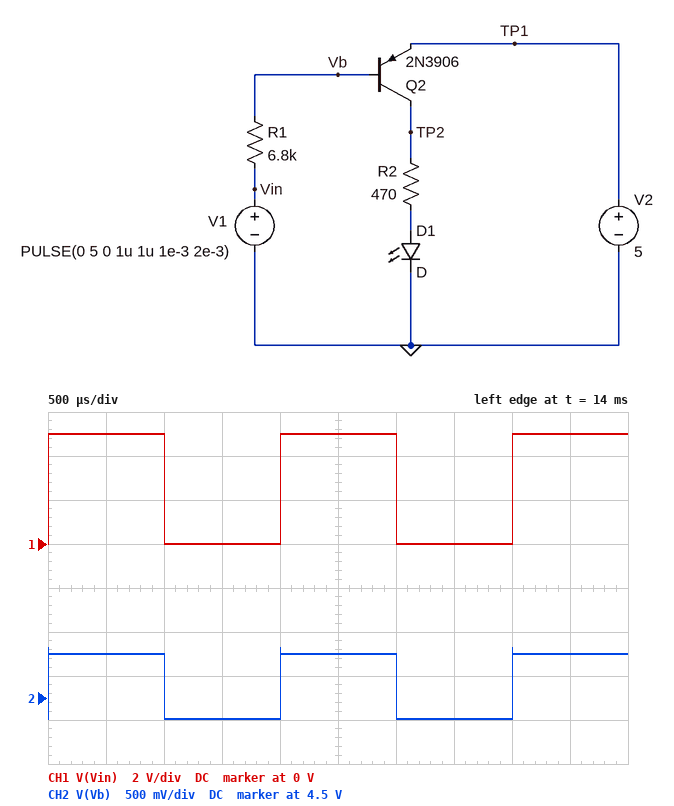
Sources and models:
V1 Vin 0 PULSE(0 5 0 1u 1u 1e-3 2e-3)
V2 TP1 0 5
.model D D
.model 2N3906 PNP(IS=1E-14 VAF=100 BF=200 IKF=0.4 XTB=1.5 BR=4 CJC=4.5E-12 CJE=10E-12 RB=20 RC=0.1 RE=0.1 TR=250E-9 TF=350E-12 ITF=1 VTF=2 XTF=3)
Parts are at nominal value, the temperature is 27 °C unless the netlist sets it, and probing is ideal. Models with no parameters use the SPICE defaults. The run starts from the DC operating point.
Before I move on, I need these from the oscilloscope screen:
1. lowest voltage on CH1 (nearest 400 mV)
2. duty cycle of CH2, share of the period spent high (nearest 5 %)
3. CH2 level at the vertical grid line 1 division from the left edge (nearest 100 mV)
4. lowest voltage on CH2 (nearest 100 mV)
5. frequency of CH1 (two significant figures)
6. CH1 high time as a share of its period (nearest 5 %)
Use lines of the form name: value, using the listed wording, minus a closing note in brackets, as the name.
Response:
lowest voltage on CH1: 0 V
duty cycle of CH2, share of the period spent high: 50 %
CH2 level at the vertical grid line 1 division from the left edge: 5.0 V
lowest voltage on CH2: 4.3 V
frequency of CH1: 500 Hz
CH1 high time as a share of its period: 50 %
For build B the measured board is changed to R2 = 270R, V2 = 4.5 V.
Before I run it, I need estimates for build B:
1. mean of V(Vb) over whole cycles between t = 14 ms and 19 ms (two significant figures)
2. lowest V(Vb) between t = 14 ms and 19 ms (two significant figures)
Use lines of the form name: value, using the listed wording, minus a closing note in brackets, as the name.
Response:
mean of V(Vb) over whole cycles between t = 14 ms and 19 ms: 4.4 V
lowest V(Vb) between t = 14 ms and 19 ms: 3.8 V
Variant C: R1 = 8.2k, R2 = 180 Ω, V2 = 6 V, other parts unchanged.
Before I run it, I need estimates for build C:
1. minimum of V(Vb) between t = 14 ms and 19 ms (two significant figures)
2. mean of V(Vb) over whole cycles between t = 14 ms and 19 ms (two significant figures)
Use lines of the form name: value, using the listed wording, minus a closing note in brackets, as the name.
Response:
minimum of V(Vb) between t = 14 ms and 19 ms: 5.2 V
mean of V(Vb) over whole cycles between t = 14 ms and 19 ms: 5.3 V
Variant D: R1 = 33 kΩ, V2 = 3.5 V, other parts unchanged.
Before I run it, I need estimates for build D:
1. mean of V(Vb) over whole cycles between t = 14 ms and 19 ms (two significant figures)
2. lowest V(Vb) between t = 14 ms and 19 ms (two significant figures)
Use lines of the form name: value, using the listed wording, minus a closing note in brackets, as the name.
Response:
mean of V(Vb) over whole cycles between t = 14 ms and 19 ms: 3.9 V
lowest V(Vb) between t = 14 ms and 19 ms: 2.8 V
